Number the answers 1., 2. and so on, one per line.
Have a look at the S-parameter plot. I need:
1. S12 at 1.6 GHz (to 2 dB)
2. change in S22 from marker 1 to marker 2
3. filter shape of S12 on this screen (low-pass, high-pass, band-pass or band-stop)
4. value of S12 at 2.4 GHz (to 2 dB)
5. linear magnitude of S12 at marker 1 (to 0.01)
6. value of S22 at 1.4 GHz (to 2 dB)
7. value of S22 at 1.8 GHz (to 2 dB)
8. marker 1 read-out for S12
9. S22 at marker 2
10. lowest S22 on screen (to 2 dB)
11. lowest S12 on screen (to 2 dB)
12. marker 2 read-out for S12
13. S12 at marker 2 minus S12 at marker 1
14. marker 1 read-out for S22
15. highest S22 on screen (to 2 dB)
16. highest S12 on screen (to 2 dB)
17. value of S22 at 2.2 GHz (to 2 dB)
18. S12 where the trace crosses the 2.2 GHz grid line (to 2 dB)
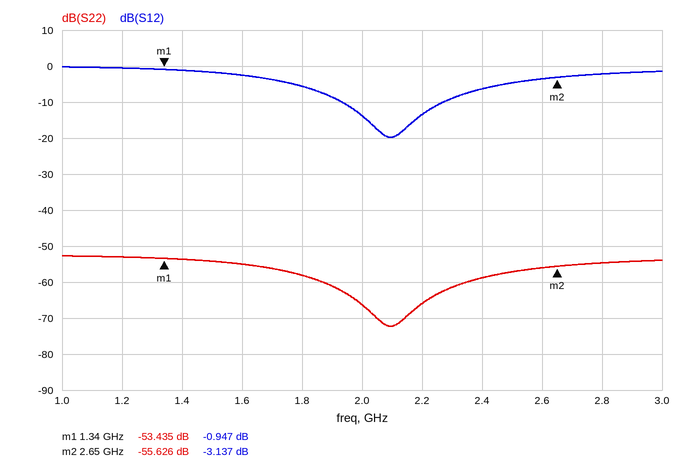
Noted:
1. -2 dB
2. -2.191 dB
3. band-stop
4. -6 dB
5. 0.90
6. -54 dB
7. -58 dB
8. -0.947 dB
9. -55.626 dB
10. -72 dB
11. -20 dB
12. -3.137 dB
13. -2.190 dB
14. -53.435 dB
15. -52 dB
16. 0 dB
17. -66 dB
18. -14 dB
